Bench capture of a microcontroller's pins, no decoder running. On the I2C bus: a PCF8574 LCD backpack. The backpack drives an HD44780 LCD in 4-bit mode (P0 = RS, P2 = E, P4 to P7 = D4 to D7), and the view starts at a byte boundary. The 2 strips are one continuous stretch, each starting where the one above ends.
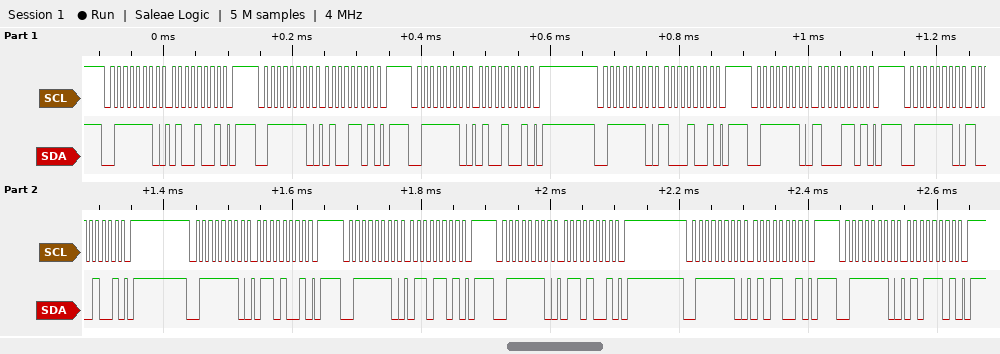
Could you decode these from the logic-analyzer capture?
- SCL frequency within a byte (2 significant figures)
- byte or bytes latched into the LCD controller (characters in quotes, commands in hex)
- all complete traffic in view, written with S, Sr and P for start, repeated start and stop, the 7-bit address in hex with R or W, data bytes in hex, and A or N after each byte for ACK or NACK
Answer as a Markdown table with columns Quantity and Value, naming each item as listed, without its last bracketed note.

| Quantity | Value |
|---|---|
| SCL frequency within a byte | 100 kHz |
| byte or bytes latched into the LCD controller | 'H' |
| all complete traffic in view, written with S, Sr and P for start, repeated start and stop, the 7-bit address in hex with R or W, data bytes in hex, and A or N after each byte for ACK or NACK | S 3FW A 49 A P S 3FW A 4D A P S 3FW A 49 A P S 3FW A 89 A P S 3FW A 8D A P S 3FW A 89 A P S 3FW A 69 A P S 3FW A 6D A P S 3FW A 69 A P S 3FW A 59 A P S 3FW A 5D A P |
